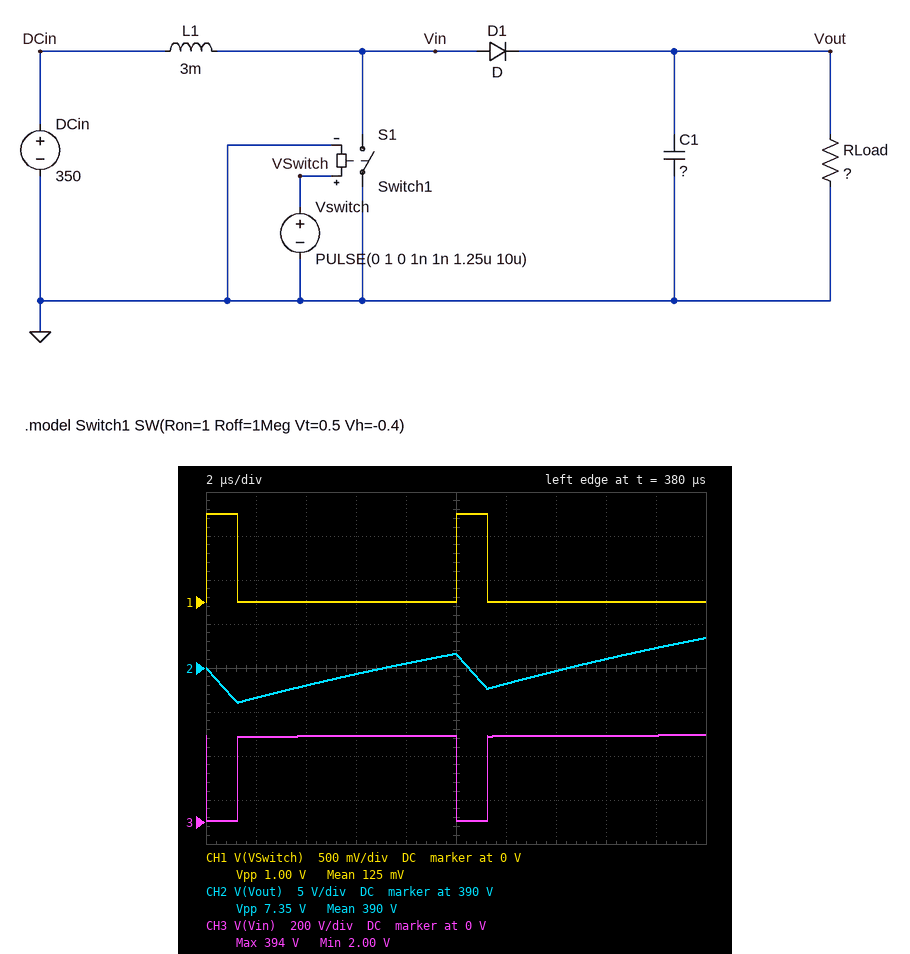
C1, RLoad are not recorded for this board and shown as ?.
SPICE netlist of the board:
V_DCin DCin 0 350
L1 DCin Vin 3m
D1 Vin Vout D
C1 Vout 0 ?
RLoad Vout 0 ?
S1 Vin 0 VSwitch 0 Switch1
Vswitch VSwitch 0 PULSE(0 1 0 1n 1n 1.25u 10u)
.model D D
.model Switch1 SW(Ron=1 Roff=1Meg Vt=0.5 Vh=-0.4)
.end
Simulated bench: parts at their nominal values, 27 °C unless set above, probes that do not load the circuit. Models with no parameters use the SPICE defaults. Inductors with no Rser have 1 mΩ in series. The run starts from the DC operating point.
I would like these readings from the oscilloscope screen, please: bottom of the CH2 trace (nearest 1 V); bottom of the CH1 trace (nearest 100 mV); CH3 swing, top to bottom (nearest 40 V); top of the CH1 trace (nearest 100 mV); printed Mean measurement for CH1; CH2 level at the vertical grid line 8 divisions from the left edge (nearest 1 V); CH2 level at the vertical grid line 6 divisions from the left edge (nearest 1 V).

386 V
0 V
400 V
1.0 V
125 mV
391 V
388 V
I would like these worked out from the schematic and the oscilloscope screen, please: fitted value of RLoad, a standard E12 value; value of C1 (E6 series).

180 Ω
680 nF
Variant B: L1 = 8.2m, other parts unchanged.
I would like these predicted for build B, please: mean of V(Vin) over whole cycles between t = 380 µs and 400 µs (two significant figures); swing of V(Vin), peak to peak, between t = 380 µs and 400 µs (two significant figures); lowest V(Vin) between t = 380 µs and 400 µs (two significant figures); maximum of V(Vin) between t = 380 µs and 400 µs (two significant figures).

360 V
410 V
2.5 V
420 V
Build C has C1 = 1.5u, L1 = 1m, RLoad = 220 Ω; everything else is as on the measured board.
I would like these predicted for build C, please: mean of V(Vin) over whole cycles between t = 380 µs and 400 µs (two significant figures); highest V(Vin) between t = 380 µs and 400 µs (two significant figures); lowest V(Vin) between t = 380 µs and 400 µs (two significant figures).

370 V
420 V
2.4 V
